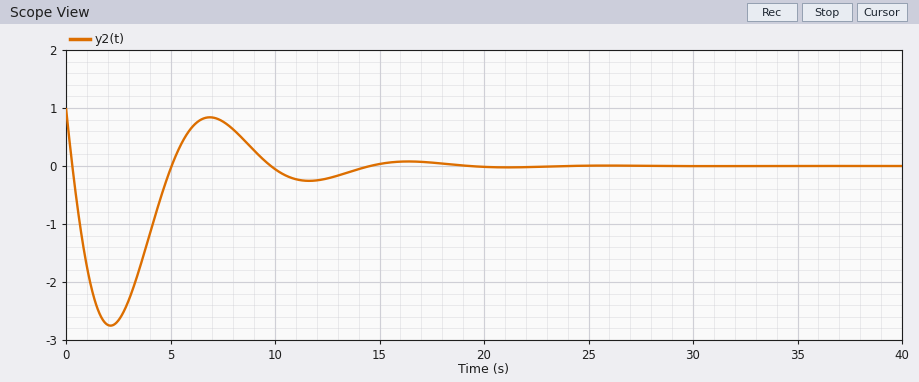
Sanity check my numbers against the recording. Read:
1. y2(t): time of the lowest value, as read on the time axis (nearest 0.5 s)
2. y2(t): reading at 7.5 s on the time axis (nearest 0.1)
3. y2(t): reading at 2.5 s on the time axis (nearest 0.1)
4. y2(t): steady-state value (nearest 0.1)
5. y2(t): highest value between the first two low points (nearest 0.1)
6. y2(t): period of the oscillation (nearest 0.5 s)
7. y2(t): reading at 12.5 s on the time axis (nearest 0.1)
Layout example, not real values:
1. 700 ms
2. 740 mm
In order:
1. 2.0 s
2. 0.8
3. -2.7
4. 0.0
5. 0.8
6. 9.5 s
7. -0.2
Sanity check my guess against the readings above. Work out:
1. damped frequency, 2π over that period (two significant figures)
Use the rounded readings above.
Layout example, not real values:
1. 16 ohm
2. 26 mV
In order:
1. 0.66 rad/s
